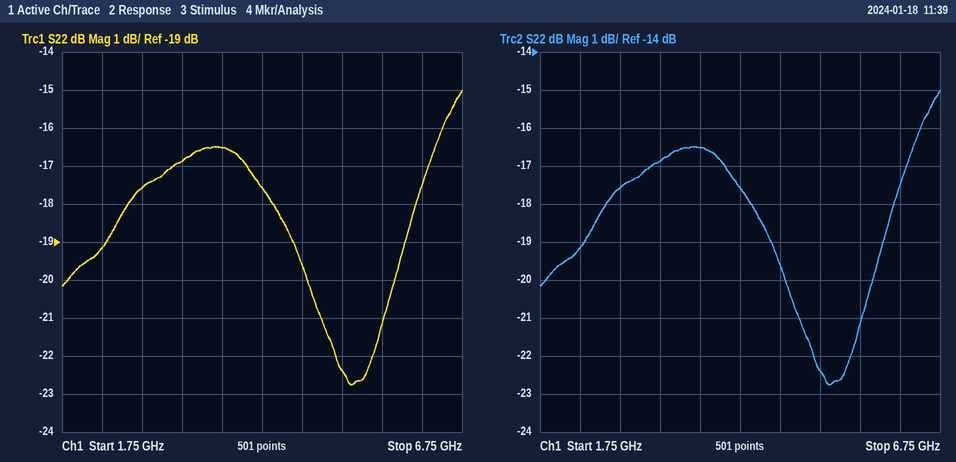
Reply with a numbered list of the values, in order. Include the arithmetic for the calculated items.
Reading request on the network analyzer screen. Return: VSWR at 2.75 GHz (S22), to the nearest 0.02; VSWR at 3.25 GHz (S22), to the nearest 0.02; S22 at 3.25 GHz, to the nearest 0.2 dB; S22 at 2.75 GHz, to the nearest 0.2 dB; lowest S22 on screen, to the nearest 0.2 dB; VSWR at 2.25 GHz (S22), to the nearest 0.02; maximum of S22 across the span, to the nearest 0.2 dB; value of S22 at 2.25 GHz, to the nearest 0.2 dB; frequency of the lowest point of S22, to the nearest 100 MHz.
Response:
1. |Γ| = 10^(-17.6/20) = 0.1318; VSWR = (1 + 0.1318)/(1 − 0.1318) ≈ 1.30
2. |Γ| = 10^(-16.8/20) = 0.1445; VSWR = (1 + 0.1445)/(1 − 0.1445) ≈ 1.34
3. -16.8 dB
4. -17.6 dB
5. -22.8 dB
6. |Γ| = 10^(-19.2/20) = 0.1096; VSWR = (1 + 0.1096)/(1 − 0.1096) ≈ 1.25, so 1.24 to the nearest 0.02
7. -15.0 dB
8. -19.2 dB
9. 5.4 GHz
